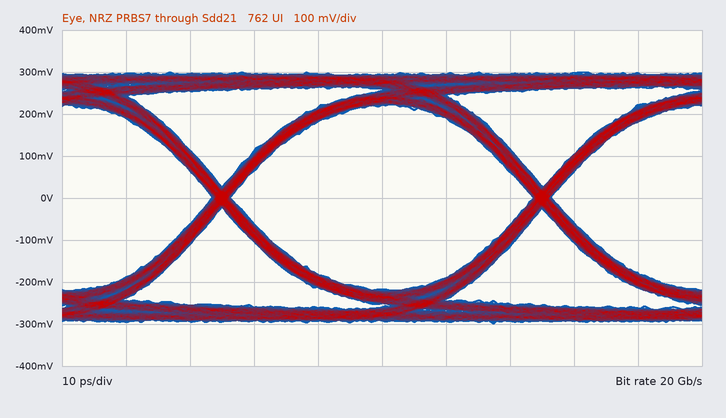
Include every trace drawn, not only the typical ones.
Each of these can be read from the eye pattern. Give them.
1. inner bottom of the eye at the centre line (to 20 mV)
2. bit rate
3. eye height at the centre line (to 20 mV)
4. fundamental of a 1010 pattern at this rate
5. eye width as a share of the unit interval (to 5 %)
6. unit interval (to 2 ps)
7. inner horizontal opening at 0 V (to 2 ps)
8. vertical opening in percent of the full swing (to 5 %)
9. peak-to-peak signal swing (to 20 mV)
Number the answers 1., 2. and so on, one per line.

1. -220 mV
2. 20 Gb/s
3. 440 mV
4. 10 GHz
5. 95 %
6. 50 ps
7. 48 ps
8. 75 %
9. 600 mV
